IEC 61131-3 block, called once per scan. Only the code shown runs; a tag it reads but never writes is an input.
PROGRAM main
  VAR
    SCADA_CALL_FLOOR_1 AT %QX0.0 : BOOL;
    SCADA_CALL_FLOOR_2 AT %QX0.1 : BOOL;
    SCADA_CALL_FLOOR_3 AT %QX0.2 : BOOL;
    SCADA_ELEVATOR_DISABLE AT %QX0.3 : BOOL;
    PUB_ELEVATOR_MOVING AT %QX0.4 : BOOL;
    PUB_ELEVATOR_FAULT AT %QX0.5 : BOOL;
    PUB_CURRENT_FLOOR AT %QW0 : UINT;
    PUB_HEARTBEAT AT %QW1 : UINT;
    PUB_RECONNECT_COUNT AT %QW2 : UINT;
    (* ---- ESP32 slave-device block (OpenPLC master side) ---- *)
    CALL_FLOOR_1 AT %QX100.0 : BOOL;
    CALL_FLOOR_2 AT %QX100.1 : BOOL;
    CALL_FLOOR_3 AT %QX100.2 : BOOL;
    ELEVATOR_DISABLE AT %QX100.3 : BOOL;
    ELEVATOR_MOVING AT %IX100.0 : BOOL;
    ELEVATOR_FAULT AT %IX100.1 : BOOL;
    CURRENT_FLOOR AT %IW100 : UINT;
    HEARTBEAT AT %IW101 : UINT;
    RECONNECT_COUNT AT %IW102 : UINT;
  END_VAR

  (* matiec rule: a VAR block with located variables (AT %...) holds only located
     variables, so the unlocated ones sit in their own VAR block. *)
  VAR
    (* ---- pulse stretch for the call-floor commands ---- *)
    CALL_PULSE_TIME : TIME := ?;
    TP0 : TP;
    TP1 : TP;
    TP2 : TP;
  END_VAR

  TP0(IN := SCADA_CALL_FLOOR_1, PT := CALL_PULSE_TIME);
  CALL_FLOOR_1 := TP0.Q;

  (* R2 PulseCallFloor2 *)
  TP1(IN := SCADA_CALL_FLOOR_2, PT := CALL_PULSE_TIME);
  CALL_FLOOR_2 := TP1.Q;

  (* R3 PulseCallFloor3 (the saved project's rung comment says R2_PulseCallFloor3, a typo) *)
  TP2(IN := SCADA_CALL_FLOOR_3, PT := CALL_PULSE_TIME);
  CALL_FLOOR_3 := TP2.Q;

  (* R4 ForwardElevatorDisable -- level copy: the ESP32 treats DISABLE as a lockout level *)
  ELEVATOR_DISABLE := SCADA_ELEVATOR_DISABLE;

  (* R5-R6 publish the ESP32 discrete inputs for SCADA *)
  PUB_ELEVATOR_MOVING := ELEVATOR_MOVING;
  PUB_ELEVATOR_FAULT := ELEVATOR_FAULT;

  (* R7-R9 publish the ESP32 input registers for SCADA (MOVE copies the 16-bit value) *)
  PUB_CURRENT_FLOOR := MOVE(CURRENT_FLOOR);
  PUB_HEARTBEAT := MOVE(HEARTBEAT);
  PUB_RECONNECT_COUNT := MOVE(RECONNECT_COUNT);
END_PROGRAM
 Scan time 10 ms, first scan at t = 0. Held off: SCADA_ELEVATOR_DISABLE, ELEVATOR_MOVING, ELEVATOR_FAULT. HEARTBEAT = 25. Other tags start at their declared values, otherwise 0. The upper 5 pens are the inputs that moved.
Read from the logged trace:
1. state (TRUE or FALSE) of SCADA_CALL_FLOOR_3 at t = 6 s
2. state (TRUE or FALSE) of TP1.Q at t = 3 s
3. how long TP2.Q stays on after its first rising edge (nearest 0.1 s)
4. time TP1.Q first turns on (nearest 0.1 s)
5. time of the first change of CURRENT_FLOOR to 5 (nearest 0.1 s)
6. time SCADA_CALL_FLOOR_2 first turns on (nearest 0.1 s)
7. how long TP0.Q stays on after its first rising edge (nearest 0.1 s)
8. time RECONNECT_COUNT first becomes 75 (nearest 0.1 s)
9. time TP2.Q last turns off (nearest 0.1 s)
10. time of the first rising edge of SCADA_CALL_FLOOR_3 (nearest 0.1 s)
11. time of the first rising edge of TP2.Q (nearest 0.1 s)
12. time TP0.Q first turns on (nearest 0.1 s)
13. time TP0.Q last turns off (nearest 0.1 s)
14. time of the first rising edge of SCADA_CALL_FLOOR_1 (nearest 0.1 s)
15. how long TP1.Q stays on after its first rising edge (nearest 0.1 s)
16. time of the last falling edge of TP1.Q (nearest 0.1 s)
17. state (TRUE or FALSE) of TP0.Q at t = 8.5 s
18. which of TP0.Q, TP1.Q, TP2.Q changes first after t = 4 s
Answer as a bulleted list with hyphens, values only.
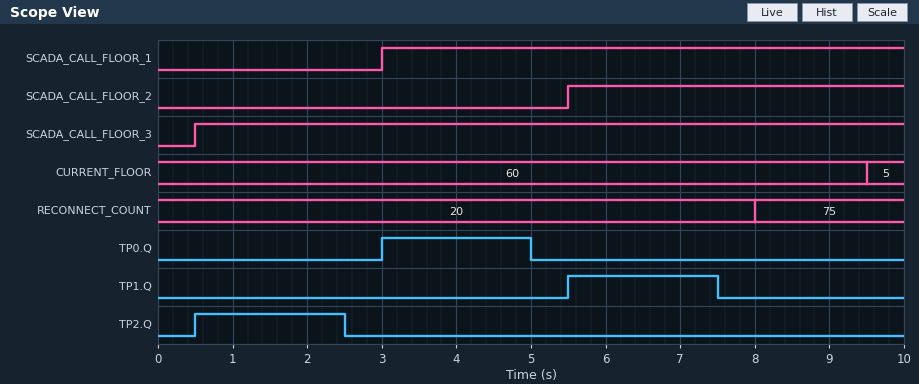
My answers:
- TRUE
- FALSE
- 2.0 s
- 5.5 s
- 9.5 s
- 5.5 s
- 2.0 s
- 8.0 s
- 2.5 s
- 0.5 s
- 0.5 s
- 3.0 s
- 5.0 s
- 3.0 s
- 2.0 s
- 7.5 s
- FALSE
- TP0.Q
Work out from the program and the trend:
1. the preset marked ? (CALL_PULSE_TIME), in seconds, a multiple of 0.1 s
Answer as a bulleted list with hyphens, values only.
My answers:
- 2.0 s
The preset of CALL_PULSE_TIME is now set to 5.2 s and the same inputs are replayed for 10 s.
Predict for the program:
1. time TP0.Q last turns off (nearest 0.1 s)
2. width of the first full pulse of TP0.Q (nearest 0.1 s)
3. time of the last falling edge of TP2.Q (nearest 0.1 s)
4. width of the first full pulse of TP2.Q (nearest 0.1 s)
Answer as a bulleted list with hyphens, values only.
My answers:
- 8.2 s
- 5.2 s
- 5.7 s
- 5.2 s
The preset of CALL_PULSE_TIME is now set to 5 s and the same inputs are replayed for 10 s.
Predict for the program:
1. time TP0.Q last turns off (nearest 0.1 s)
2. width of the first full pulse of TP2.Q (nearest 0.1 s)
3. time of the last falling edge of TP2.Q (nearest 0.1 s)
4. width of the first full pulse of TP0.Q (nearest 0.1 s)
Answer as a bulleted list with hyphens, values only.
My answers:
- 8.0 s
- 5.0 s
- 5.5 s
- 5.0 s
